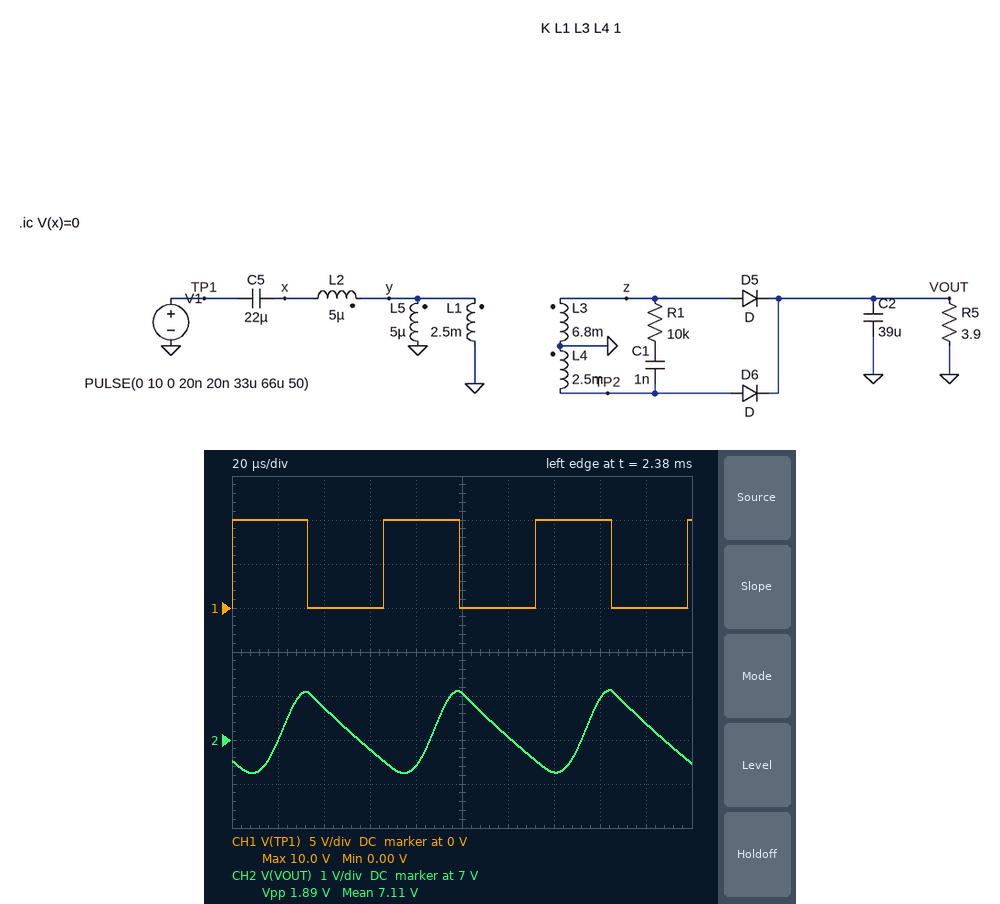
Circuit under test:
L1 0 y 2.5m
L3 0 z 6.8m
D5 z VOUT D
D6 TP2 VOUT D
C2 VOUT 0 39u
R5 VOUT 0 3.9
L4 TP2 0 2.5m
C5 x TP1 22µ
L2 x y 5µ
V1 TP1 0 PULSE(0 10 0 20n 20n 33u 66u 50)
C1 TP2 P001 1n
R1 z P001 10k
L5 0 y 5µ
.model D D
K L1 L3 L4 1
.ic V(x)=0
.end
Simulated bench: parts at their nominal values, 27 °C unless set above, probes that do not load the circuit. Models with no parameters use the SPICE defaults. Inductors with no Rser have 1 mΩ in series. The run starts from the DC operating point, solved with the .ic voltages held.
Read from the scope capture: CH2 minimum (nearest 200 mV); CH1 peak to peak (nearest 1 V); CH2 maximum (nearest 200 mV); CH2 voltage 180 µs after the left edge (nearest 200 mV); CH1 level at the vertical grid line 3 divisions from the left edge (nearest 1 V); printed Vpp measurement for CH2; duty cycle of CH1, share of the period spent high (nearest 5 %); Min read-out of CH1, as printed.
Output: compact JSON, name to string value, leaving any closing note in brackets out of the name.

{"CH2 minimum": "6.2 V", "CH1 peak to peak": "10 V", "CH2 maximum": "8.2 V", "CH2 voltage 180 µs after the left edge": "7.4 V", "CH1 level at the vertical grid line 3 divisions from the left edge": "0 V", "printed Vpp measurement for CH2": "1.89 V", "duty cycle of CH1, share of the period spent high": "50 %", "Min read-out of CH1, as printed": "0.00 V"}
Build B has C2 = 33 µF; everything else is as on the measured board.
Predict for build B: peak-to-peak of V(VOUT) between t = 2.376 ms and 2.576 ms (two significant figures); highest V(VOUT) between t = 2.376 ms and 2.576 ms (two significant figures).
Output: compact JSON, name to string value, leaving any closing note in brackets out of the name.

{"peak-to-peak of V(VOUT) between t = 2.376 ms and 2.576 ms": "2.2 V", "highest V(VOUT) between t = 2.376 ms and 2.576 ms": "8.4 V"}
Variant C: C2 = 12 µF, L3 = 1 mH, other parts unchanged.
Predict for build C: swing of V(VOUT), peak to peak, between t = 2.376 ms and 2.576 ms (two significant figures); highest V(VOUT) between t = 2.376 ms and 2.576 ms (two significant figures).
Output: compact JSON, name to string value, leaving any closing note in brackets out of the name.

{"swing of V(VOUT), peak to peak, between t = 2.376 ms and 2.576 ms": "3.9 V", "highest V(VOUT) between t = 2.376 ms and 2.576 ms": "6.3 V"}
